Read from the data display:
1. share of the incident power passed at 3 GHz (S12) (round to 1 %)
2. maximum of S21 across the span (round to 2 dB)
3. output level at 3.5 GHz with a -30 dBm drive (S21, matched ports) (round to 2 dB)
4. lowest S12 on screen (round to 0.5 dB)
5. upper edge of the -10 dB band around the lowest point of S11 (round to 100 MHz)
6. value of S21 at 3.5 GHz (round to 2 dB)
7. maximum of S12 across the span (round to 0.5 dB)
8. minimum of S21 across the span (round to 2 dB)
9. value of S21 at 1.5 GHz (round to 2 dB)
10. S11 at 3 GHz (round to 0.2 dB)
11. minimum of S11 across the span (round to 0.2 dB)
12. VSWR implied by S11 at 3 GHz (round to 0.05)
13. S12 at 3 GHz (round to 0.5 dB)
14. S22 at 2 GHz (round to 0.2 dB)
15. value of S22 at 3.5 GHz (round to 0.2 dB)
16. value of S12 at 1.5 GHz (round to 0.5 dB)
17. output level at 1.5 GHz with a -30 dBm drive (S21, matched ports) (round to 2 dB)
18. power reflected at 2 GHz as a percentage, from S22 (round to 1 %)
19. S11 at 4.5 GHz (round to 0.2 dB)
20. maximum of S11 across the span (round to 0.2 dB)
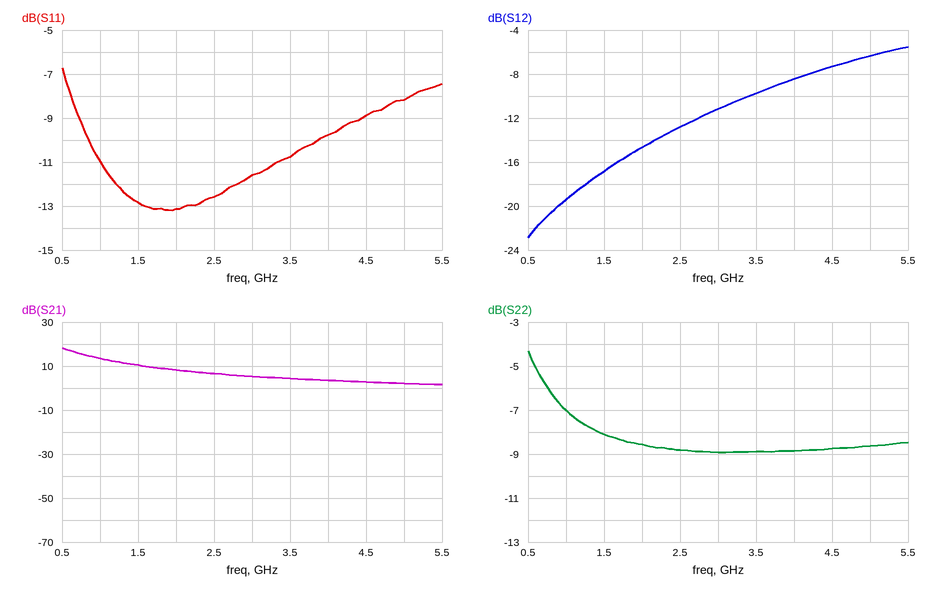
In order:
8 %
18 dB
-26 dBm
-23.0 dB
3.9 GHz
4 dB
-5.5 dB
2 dB
10 dB
-11.6 dB
-13.2 dB
1.70
-11.0 dB
-8.6 dB
-8.8 dB
-17.0 dB
-20 dBm
14 %
-8.8 dB
-6.8 dB
